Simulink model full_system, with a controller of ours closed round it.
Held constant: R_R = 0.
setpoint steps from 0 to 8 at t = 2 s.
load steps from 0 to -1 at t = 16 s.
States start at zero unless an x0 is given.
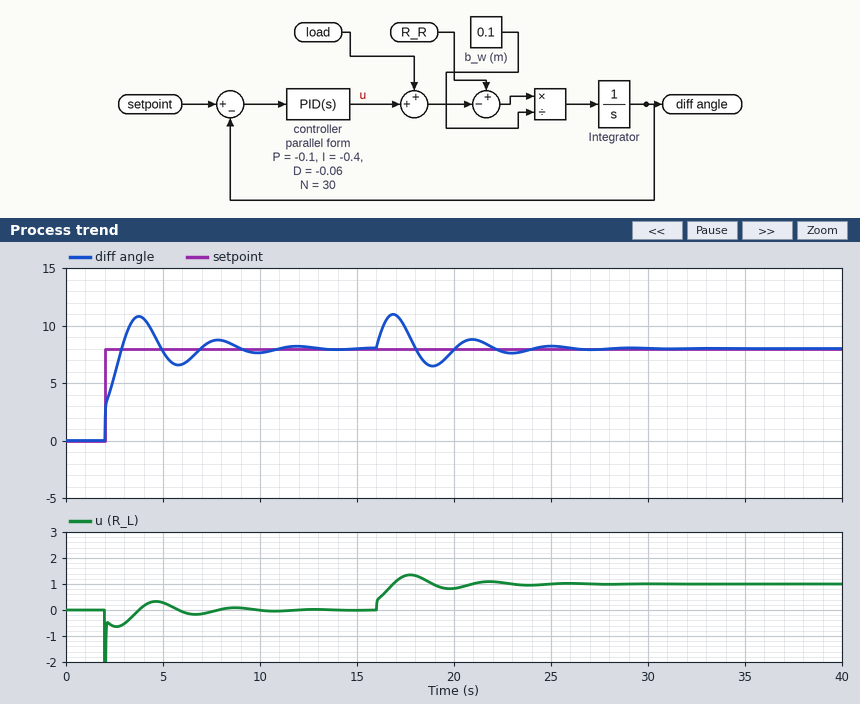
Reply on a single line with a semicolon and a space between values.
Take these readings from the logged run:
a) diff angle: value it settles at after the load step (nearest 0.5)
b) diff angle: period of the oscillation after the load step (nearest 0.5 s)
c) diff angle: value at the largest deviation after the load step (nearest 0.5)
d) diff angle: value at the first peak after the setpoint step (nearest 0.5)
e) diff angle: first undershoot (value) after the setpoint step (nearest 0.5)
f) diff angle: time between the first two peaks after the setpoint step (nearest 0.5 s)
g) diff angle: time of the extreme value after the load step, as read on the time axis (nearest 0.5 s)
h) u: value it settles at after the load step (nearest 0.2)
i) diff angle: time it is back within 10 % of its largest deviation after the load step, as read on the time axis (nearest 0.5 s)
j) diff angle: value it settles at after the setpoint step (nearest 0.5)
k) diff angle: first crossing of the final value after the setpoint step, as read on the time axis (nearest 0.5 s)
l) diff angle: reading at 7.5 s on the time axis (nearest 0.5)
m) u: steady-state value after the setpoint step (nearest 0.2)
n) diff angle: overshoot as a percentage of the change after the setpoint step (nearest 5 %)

8.0; 4.0 s; 11.0; 11.0; 6.5; 4.0 s; 17.0 s; 1.0; 23.5 s; 8.0; 3.0 s; 8.5; 0.0; 35 %
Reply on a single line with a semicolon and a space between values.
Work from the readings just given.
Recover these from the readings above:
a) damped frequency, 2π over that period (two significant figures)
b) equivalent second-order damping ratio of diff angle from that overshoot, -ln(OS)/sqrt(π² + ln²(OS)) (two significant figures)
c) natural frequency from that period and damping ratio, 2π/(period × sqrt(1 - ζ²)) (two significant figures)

1.6 rad/s; 0.32; 1.7 rad/s
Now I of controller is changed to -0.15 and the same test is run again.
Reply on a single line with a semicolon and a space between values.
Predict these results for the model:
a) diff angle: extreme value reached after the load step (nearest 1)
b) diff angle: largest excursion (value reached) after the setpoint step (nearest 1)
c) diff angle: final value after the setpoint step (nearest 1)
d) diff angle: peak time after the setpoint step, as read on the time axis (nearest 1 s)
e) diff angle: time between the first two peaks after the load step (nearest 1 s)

12; 10; 8; 5 s; 7 s
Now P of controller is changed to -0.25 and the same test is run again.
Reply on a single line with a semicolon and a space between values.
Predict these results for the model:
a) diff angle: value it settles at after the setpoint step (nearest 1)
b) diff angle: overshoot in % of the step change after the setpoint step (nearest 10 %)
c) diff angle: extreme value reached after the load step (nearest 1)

8; 20 %; 10
